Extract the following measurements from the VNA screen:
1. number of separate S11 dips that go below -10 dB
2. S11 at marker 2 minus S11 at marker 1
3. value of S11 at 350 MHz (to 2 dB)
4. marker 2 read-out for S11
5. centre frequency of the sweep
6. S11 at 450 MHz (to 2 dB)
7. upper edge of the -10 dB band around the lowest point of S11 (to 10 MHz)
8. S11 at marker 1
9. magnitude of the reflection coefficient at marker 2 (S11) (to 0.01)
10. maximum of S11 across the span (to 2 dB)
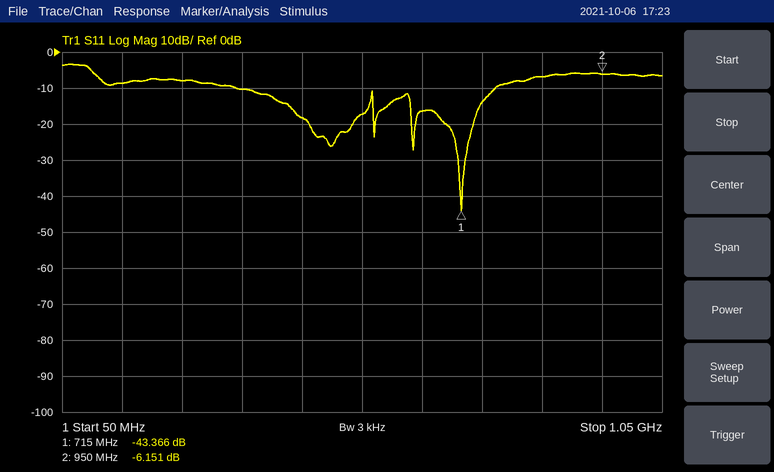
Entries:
4
37.215 dB
-10 dB
-6.151 dB
550 MHz
-18 dB
770 MHz
-43.366 dB
0.49
-4 dB
